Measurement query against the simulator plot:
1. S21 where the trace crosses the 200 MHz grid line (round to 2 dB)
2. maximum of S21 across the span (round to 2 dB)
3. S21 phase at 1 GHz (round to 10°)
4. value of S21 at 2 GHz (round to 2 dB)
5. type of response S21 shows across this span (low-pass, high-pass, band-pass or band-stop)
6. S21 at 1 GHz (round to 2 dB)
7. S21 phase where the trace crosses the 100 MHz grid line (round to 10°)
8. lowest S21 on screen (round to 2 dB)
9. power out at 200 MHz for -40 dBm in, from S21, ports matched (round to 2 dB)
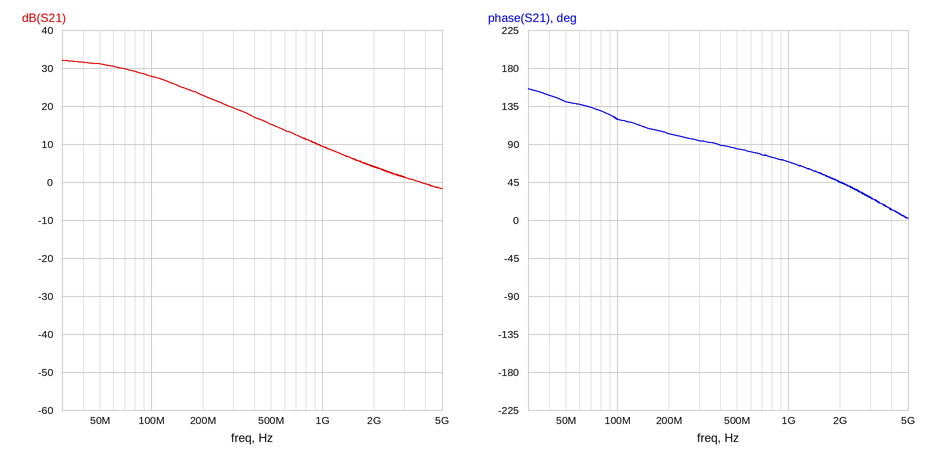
22 dB
32 dB
70°
4 dB
low-pass
10 dB
120°
-2 dB
-18 dBm
